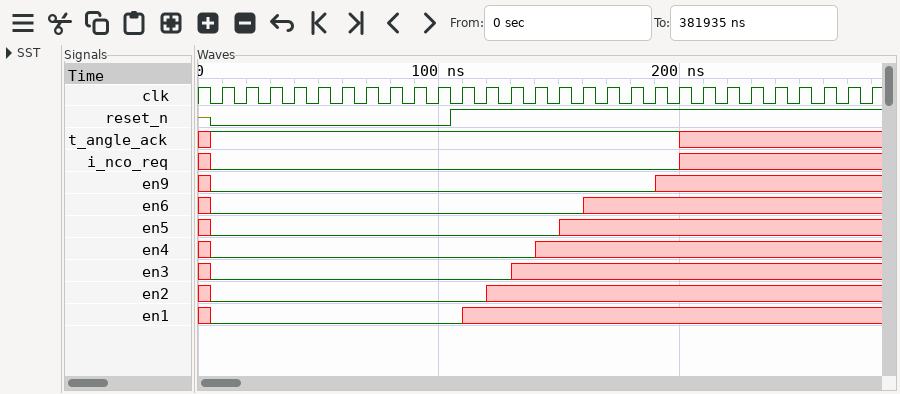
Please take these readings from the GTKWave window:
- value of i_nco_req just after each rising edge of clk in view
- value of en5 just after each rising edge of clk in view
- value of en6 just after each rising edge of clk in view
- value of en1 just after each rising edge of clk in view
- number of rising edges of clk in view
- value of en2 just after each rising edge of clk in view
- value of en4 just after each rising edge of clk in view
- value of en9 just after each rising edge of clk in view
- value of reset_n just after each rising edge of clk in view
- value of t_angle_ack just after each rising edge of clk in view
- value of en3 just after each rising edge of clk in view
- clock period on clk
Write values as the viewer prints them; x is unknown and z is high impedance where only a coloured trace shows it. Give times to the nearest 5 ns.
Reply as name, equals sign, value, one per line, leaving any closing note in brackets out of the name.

value of i_nco_req just after each rising edge of clk in view = 0 0 0 0 0 0 0 0 0 0 0 0 0 0 0 0 0 0 0 x x x x x x x x x
value of en5 just after each rising edge of clk in view = 0 0 0 0 0 0 0 0 0 0 0 0 0 0 x x x x x x x x x x x x x x
value of en6 just after each rising edge of clk in view = 0 0 0 0 0 0 0 0 0 0 0 0 0 0 0 x x x x x x x x x x x x x
value of en1 just after each rising edge of clk in view = 0 0 0 0 0 0 0 0 0 0 x x x x x x x x x x x x x x x x x x
number of rising edges of clk in view = 28
value of en2 just after each rising edge of clk in view = 0 0 0 0 0 0 0 0 0 0 0 x x x x x x x x x x x x x x x x x
value of en4 just after each rising edge of clk in view = 0 0 0 0 0 0 0 0 0 0 0 0 0 x x x x x x x x x x x x x x x
value of en9 just after each rising edge of clk in view = 0 0 0 0 0 0 0 0 0 0 0 0 0 0 0 0 0 0 x x x x x x x x x x
value of reset_n just after each rising edge of clk in view = 0 0 0 0 0 0 0 0 0 0 1 1 1 1 1 1 1 1 1 1 1 1 1 1 1 1 1 1
value of t_angle_ack just after each rising edge of clk in view = 1 1 1 1 1 1 1 1 1 1 1 1 1 1 1 1 1 1 1 x x x x x x x x x
value of en3 just after each rising edge of clk in view = 0 0 0 0 0 0 0 0 0 0 0 0 x x x x x x x x x x x x x x x x
clock period on clk = 10 ns
